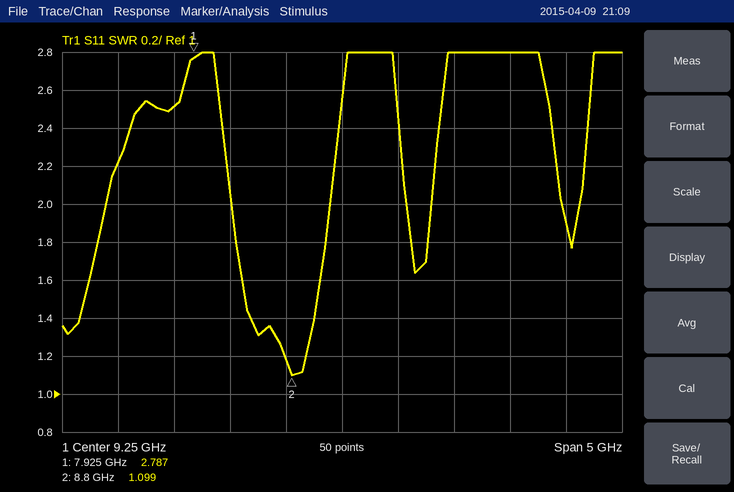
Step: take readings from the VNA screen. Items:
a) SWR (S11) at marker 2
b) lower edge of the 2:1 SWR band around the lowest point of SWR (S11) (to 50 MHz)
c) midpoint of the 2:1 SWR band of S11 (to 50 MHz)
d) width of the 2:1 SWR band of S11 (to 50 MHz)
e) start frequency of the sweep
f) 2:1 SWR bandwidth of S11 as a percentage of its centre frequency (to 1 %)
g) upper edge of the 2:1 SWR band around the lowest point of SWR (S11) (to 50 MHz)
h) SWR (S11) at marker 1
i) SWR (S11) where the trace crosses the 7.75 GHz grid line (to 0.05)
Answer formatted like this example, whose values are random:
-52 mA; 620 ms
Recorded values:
1.099; 8.25 GHz; 8.70 GHz; 900 MHz; 6.75 GHz; 10 %; 9.15 GHz; 2.787; 2.50
